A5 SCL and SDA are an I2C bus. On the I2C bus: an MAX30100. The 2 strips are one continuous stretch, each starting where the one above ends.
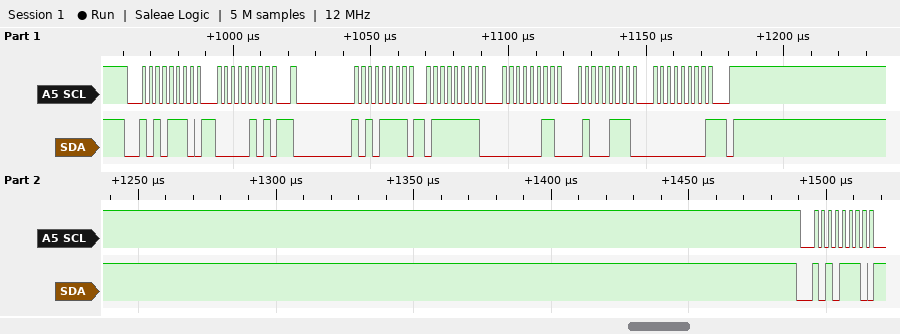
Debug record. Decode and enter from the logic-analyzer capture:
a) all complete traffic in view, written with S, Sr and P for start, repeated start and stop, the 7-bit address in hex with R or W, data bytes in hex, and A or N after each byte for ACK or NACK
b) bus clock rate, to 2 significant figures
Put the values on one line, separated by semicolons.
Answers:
S 57W A 05 A Sr 57R A 7F A 03 A 47 A 00 N P S 57W A; 400 kHz
